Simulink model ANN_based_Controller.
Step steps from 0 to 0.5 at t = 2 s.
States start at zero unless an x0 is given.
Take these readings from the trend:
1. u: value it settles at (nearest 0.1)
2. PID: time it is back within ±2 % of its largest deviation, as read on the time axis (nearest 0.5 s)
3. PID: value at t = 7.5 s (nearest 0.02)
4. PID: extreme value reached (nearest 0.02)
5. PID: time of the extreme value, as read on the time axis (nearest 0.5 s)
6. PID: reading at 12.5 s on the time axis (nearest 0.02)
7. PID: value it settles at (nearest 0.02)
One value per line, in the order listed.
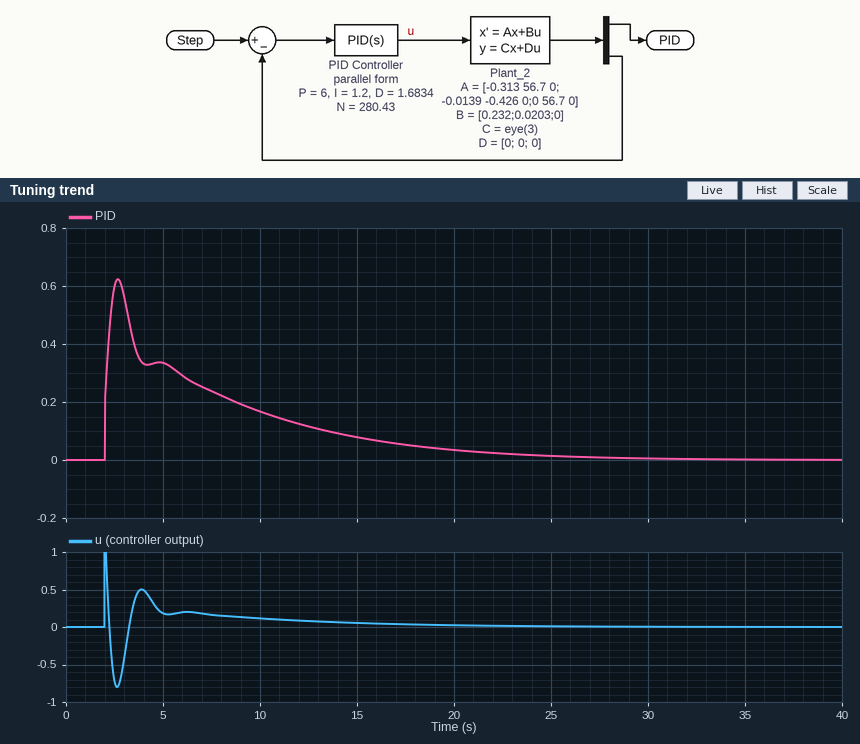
0.0
25.5 s
0.24
0.62
2.5 s
0.12
0.00
